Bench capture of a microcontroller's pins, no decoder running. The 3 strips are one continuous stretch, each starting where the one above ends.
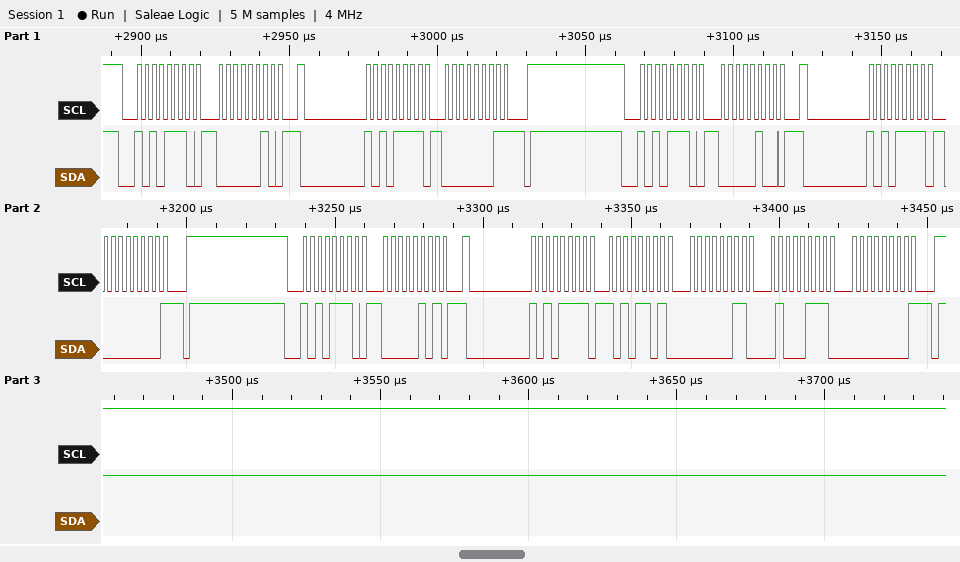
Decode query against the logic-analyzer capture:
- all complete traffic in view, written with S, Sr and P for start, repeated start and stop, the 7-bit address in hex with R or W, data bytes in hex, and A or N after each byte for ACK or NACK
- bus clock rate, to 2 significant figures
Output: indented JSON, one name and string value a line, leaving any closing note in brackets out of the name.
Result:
{
  "all complete traffic in view, written with S, Sr and P for start, repeated start and stop, the 7-bit address in hex with R or W, data bytes in hex, and A or N after each byte for ACK or NACK": "S 57W A 02 A Sr 57R A 01 N P S 57W A 04 A Sr 57R A 00 N P S 57W A 05 A Sr 57R A AD A 03 A 47 A 00 N P",
  "bus clock rate, to 2 significant figures": "400 kHz"
}
